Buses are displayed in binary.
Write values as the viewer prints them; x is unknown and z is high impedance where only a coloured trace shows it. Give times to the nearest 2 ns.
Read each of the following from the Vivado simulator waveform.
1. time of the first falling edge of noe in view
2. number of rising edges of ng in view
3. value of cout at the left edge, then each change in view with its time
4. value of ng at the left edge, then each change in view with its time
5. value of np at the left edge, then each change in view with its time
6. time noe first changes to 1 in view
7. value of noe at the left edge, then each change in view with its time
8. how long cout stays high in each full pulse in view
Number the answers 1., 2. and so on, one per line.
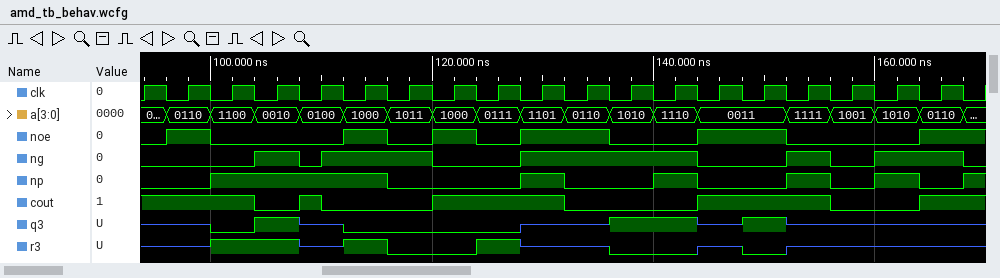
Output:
1. 100 ns
2. 5
3. 1, 0 at 104 ns, 1 at 108 ns, 0 at 110 ns, 1 at 120 ns, 0 at 132 ns, 1 at 144 ns, 0 at 156 ns, 1 at 164 ns
4. 0, 1 at 104 ns, 0 at 108 ns, 1 at 110 ns, 0 at 120 ns, 1 at 128 ns, 0 at 144 ns, 1 at 152 ns, 0 at 156 ns, 1 at 160 ns, 0 at 168 ns
5. 0, 1 at 100 ns, 0 at 116 ns, 1 at 128 ns, 0 at 132 ns, 1 at 140 ns, 0 at 144 ns, 1 at 152 ns, 0 at 156 ns, 1 at 160 ns, 0 at 164 ns, 1 at 168 ns
6. 96 ns
7. 0, 1 at 96 ns, 0 at 100 ns, 1 at 112 ns, 0 at 116 ns, 1 at 120 ns, 0 at 124 ns, 1 at 128 ns, 0 at 136 ns, 1 at 144 ns, 0 at 152 ns, 1 at 164 ns
8. 2 ns, 12 ns, 12 ns
